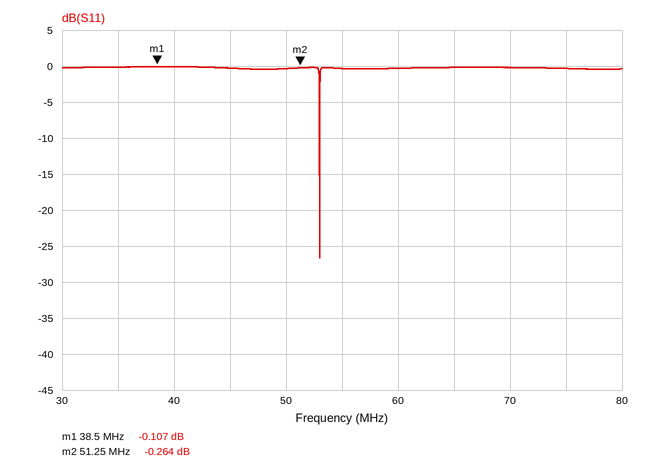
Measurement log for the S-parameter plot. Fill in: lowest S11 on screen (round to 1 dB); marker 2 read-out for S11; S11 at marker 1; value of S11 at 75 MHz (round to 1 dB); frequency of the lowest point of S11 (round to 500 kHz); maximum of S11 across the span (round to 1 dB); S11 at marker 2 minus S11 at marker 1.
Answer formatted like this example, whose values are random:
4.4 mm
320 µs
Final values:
-27 dB
-0.264 dB
-0.107 dB
0 dB
53.0 MHz
0 dB
-0.157 dB
